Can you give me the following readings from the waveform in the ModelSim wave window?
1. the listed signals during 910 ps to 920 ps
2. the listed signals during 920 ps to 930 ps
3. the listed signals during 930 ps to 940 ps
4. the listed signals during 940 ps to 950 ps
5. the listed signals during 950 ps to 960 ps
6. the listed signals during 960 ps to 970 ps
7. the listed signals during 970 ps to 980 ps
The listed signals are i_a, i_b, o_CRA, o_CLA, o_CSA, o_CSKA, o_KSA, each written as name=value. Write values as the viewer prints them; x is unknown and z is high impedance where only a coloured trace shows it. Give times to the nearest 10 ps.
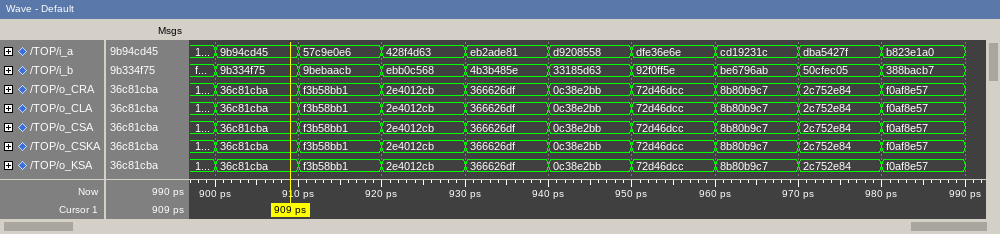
i_a=57c9e0e6, i_b=9bebaacb, o_CRA=f3b58bb1, o_CLA=f3b58bb1, o_CSA=f3b58bb1, o_CSKA=f3b58bb1, o_KSA=f3b58bb1
i_a=428f4d63, i_b=ebb0c568, o_CRA=2e4012cb, o_CLA=2e4012cb, o_CSA=2e4012cb, o_CSKA=2e4012cb, o_KSA=2e4012cb
i_a=eb2ade81, i_b=4b3b485e, o_CRA=366626df, o_CLA=366626df, o_CSA=366626df, o_CSKA=366626df, o_KSA=366626df
i_a=d9208558, i_b=33185d63, o_CRA=0c38e2bb, o_CLA=0c38e2bb, o_CSA=0c38e2bb, o_CSKA=0c38e2bb, o_KSA=0c38e2bb
i_a=dfe36e6e, i_b=92f0ff5e, o_CRA=72d46dcc, o_CLA=72d46dcc, o_CSA=72d46dcc, o_CSKA=72d46dcc, o_KSA=72d46dcc
i_a=cd19231c, i_b=be6796ab, o_CRA=8b80b9c7, o_CLA=8b80b9c7, o_CSA=8b80b9c7, o_CSKA=8b80b9c7, o_KSA=8b80b9c7
i_a=dba5427f, i_b=50cfec05, o_CRA=2c752e84, o_CLA=2c752e84, o_CSA=2c752e84, o_CSKA=2c752e84, o_KSA=2c752e84
